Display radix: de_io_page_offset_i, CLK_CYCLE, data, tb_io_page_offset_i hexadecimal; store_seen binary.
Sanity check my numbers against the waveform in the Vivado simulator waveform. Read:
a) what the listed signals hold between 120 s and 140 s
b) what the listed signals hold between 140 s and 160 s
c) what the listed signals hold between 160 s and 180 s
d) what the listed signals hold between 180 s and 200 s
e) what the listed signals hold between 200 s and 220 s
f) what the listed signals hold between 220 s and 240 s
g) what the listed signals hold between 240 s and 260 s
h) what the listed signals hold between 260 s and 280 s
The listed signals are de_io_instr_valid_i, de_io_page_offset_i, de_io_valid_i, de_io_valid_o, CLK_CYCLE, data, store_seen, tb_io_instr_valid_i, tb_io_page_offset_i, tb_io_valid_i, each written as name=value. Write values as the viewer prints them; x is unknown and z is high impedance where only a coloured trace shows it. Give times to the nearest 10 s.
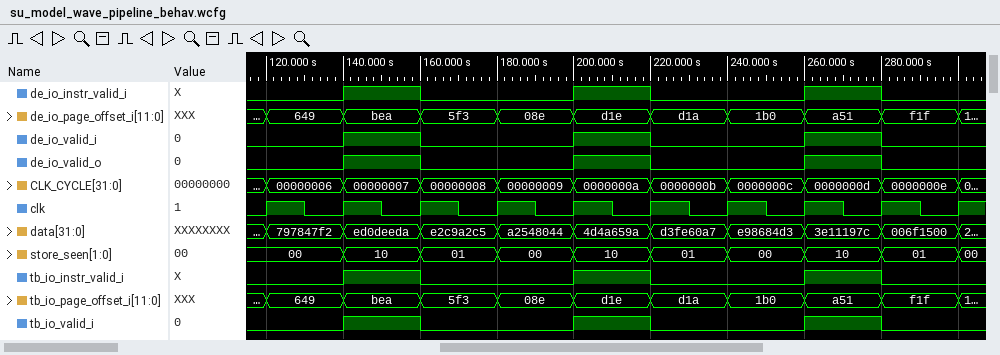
de_io_instr_valid_i=0, de_io_page_offset_i=649, de_io_valid_i=0, de_io_valid_o=0, CLK_CYCLE=00000006, data=797847f2, store_seen=00, tb_io_instr_valid_i=0, tb_io_page_offset_i=649, tb_io_valid_i=0
de_io_instr_valid_i=1, de_io_page_offset_i=bea, de_io_valid_i=1, de_io_valid_o=1, CLK_CYCLE=00000007, data=ed0deeda, store_seen=10, tb_io_instr_valid_i=1, tb_io_page_offset_i=bea, tb_io_valid_i=1
de_io_instr_valid_i=0, de_io_page_offset_i=5f3, de_io_valid_i=0, de_io_valid_o=0, CLK_CYCLE=00000008, data=e2c9a2c5, store_seen=01, tb_io_instr_valid_i=0, tb_io_page_offset_i=5f3, tb_io_valid_i=0
de_io_instr_valid_i=0, de_io_page_offset_i=08e, de_io_valid_i=0, de_io_valid_o=0, CLK_CYCLE=00000009, data=a2548044, store_seen=00, tb_io_instr_valid_i=0, tb_io_page_offset_i=08e, tb_io_valid_i=0
de_io_instr_valid_i=1, de_io_page_offset_i=d1e, de_io_valid_i=1, de_io_valid_o=1, CLK_CYCLE=0000000a, data=4d4a659a, store_seen=10, tb_io_instr_valid_i=1, tb_io_page_offset_i=d1e, tb_io_valid_i=1
de_io_instr_valid_i=0, de_io_page_offset_i=d1a, de_io_valid_i=0, de_io_valid_o=0, CLK_CYCLE=0000000b, data=d3fe60a7, store_seen=01, tb_io_instr_valid_i=0, tb_io_page_offset_i=d1a, tb_io_valid_i=0
de_io_instr_valid_i=0, de_io_page_offset_i=1b0, de_io_valid_i=0, de_io_valid_o=0, CLK_CYCLE=0000000c, data=e98684d3, store_seen=00, tb_io_instr_valid_i=0, tb_io_page_offset_i=1b0, tb_io_valid_i=0
de_io_instr_valid_i=1, de_io_page_offset_i=a51, de_io_valid_i=1, de_io_valid_o=1, CLK_CYCLE=0000000d, data=3e11197c, store_seen=10, tb_io_instr_valid_i=1, tb_io_page_offset_i=a51, tb_io_valid_i=1
